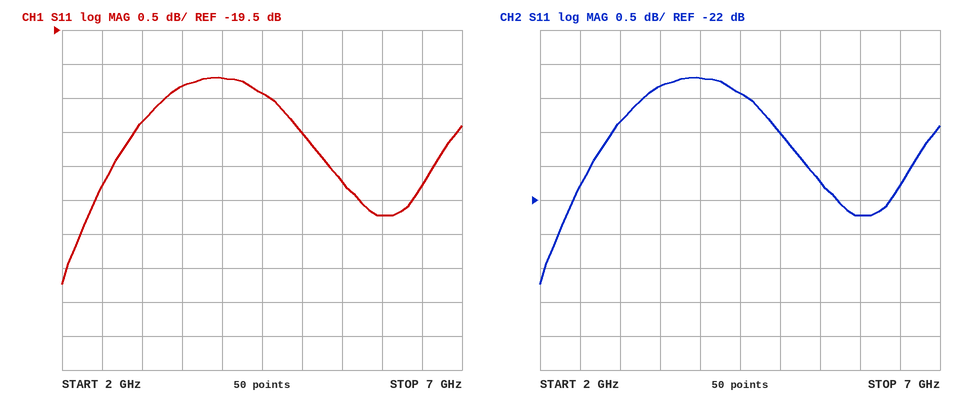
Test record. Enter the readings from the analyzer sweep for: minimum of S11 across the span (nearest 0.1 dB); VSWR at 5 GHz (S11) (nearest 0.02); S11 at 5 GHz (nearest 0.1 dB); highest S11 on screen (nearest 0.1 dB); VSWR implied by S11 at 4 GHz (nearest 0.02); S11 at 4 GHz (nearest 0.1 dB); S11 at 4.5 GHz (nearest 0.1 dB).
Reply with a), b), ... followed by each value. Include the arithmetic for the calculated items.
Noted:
a) -23.2 dB
b) |Γ| = 10^(-21/20) = 0.0891; VSWR = (1 + 0.0891)/(1 − 0.0891) ≈ 1.20
c) -21.0 dB
d) -20.2 dB
e) |Γ| = 10^(-20.2/20) = 0.0977; VSWR = (1 + 0.0977)/(1 − 0.0977) ≈ 1.22
f) -20.2 dB
g) -20.4 dB
